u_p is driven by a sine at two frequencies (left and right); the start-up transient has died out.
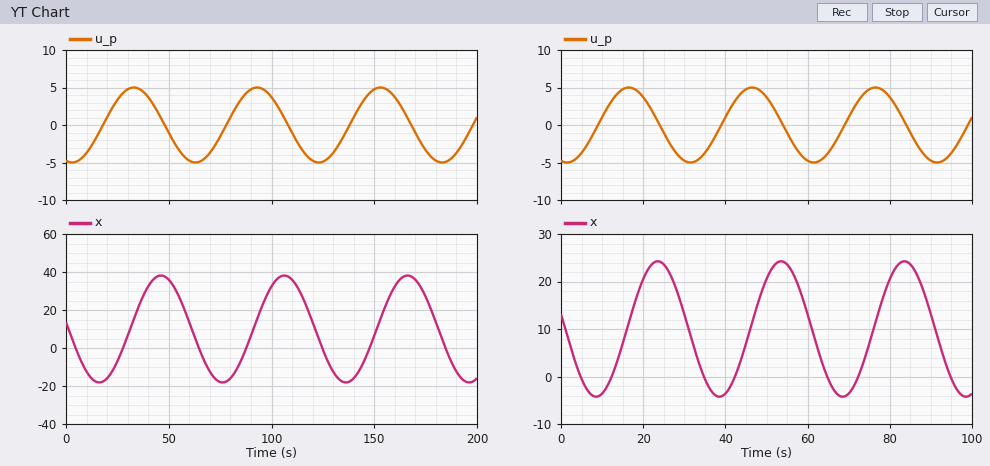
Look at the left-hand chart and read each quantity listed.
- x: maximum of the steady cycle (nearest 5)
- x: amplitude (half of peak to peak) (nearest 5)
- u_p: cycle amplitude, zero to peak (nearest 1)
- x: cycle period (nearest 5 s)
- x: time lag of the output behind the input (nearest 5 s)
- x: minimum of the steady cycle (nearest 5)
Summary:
40
30
5
60 s
15 s
-20
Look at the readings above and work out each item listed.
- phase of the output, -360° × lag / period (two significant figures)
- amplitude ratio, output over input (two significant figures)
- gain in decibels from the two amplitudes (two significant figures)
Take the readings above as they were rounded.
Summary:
-90°
6.0
16 dB
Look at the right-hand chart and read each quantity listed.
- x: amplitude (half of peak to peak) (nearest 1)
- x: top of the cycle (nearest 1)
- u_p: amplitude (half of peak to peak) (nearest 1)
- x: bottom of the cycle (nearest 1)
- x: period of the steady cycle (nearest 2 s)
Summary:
14
24
5
-4
30 s
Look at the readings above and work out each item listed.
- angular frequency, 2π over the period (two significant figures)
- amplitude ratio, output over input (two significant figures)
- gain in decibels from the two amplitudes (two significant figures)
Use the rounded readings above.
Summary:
0.21 rad/s
2.8
8.9 dB
